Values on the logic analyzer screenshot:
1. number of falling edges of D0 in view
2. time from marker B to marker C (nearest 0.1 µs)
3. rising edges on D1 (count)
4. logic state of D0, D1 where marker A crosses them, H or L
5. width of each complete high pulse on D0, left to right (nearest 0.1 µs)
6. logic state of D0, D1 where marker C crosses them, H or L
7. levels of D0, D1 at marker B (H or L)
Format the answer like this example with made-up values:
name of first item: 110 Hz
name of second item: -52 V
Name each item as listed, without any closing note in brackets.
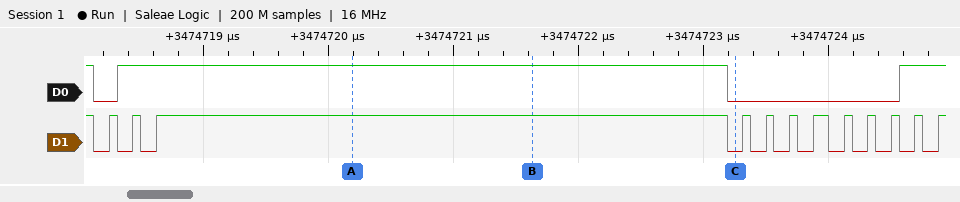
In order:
number of falling edges of D0 in view: 2
time from marker B to marker C: 1.6 µs
rising edges on D1: 12
logic state of D0, D1 where marker A crosses them, H or L: D0=H, D1=H
width of each complete high pulse on D0, left to right: 4.9 µs
logic state of D0, D1 where marker C crosses them, H or L: D0=L, D1=L
levels of D0, D1 at marker B: D0=H, D1=H
